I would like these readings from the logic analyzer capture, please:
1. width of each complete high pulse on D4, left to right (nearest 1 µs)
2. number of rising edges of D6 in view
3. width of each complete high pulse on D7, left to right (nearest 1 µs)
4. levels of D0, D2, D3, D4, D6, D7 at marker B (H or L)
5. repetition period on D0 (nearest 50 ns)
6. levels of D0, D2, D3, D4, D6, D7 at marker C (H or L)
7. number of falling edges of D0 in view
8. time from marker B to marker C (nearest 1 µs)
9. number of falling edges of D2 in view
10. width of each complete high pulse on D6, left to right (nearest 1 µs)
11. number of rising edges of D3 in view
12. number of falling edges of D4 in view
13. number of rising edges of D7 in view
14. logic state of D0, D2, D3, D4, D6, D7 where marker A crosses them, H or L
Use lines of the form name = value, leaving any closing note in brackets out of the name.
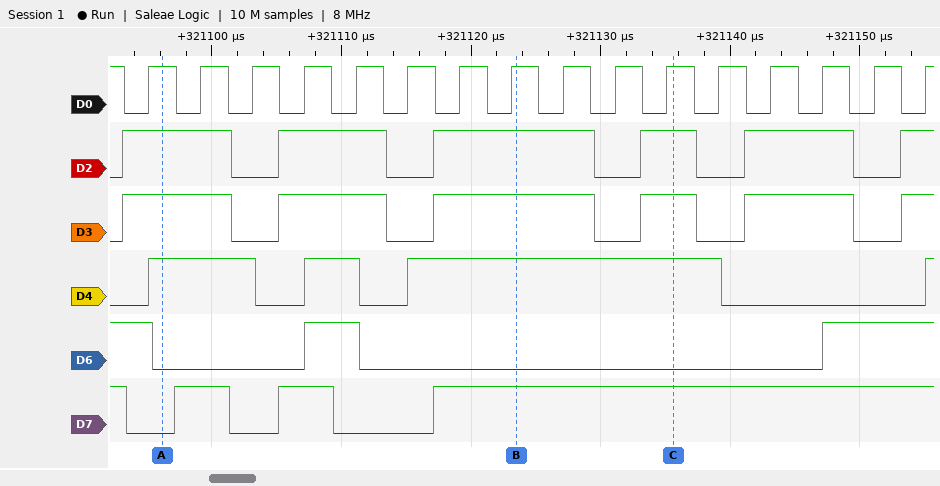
width of each complete high pulse on D4, left to right = 8 µs, 4 µs, 24 µs
number of rising edges of D6 in view = 2
width of each complete high pulse on D7, left to right = 4 µs, 4 µs
levels of D0, D2, D3, D4, D6, D7 at marker B = D0=H, D2=H, D3=H, D4=H, D6=L, D7=H
repetition period on D0 = 4000 ns
levels of D0, D2, D3, D4, D6, D7 at marker C = D0=H, D2=H, D3=H, D4=H, D6=L, D7=H
number of falling edges of D0 in view = 16
time from marker B to marker C = 12 µs
number of falling edges of D2 in view = 5
width of each complete high pulse on D6, left to right = 4 µs
number of rising edges of D3 in view = 6
number of falling edges of D4 in view = 3
number of rising edges of D7 in view = 3
logic state of D0, D2, D3, D4, D6, D7 where marker A crosses them, H or L = D0=H, D2=H, D3=H, D4=H, D6=L, D7=L
